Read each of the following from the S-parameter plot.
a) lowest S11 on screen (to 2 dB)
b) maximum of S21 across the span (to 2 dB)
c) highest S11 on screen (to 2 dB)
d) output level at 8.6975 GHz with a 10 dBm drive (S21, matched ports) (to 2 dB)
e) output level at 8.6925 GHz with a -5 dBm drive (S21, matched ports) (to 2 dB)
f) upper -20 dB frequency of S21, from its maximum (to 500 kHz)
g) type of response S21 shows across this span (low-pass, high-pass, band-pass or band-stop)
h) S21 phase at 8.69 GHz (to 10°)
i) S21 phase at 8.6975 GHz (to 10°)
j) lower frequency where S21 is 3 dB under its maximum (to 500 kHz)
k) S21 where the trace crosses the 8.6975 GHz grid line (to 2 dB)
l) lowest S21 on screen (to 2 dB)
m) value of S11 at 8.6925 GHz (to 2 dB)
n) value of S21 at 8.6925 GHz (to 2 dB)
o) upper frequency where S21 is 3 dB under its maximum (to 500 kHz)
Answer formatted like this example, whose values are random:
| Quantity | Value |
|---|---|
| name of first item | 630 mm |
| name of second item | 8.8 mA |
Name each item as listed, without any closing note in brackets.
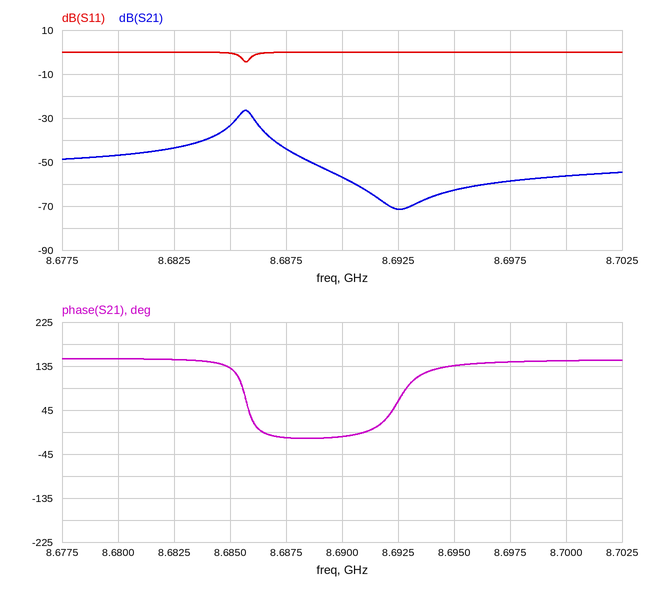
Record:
| Quantity | Value |
|---|---|
| lowest S11 on screen | -4 dB |
| maximum of S21 across the span | -26 dB |
| highest S11 on screen | 0 dB |
| output level at 8.6975 GHz with a 10 dBm drive (S21, matched ports) | -48 dBm |
| output level at 8.6925 GHz with a -5 dBm drive (S21, matched ports) | -76 dBm |
| upper -20 dB frequency of S21, from its maximum | 8.6880 GHz |
| type of response S21 shows across this span | band-pass |
| S21 phase at 8.69 GHz | -10° |
| S21 phase at 8.6975 GHz | 140° |
| lower frequency where S21 is 3 dB under its maximum | 8.6855 GHz |
| S21 where the trace crosses the 8.6975 GHz grid line | -58 dB |
| lowest S21 on screen | -72 dB |
| value of S11 at 8.6925 GHz | 0 dB |
| value of S21 at 8.6925 GHz | -72 dB |
| upper frequency where S21 is 3 dB under its maximum | 8.6860 GHz |
